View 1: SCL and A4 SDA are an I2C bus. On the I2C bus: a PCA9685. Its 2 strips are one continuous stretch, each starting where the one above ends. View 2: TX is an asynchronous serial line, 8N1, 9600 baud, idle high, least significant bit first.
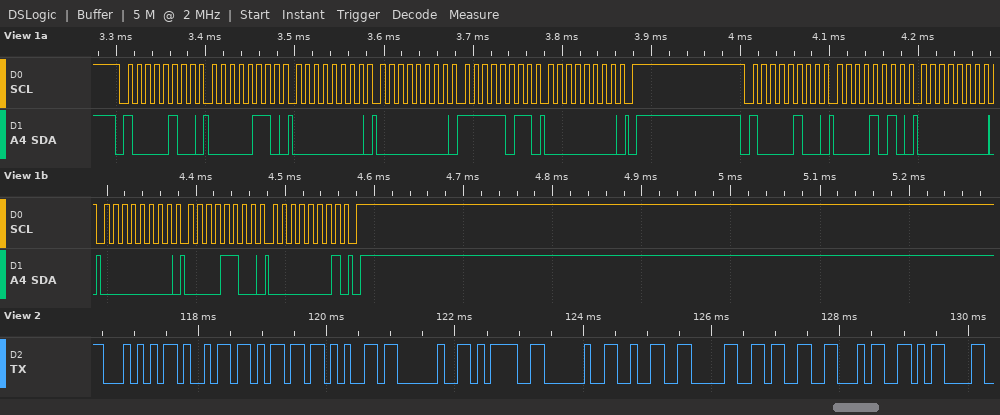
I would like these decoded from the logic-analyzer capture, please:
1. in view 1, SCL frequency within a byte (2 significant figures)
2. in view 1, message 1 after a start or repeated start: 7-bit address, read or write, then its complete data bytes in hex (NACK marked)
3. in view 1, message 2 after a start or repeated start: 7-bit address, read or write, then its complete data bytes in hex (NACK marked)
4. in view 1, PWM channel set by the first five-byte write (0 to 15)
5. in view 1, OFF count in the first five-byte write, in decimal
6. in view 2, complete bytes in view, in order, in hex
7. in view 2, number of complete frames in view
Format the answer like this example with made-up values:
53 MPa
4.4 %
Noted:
100 kHz
0x42 write: 06 00 00 FB 00
0x42 write: 0A 00 00 0C 01
0
251
0x54 0x69 0x6D 0x65 0x20 0x3D 0x20 0x32 0x30 0x33 0x34 0x0D
12
